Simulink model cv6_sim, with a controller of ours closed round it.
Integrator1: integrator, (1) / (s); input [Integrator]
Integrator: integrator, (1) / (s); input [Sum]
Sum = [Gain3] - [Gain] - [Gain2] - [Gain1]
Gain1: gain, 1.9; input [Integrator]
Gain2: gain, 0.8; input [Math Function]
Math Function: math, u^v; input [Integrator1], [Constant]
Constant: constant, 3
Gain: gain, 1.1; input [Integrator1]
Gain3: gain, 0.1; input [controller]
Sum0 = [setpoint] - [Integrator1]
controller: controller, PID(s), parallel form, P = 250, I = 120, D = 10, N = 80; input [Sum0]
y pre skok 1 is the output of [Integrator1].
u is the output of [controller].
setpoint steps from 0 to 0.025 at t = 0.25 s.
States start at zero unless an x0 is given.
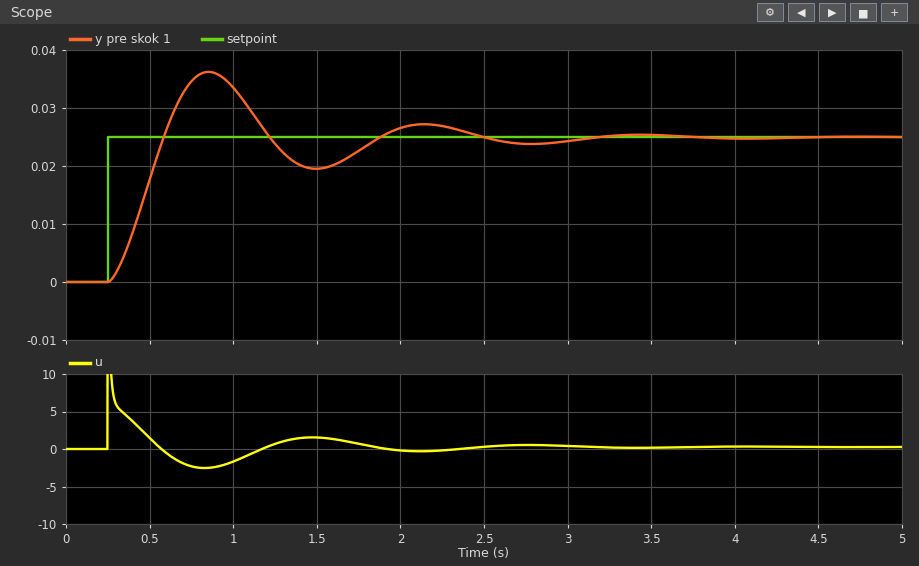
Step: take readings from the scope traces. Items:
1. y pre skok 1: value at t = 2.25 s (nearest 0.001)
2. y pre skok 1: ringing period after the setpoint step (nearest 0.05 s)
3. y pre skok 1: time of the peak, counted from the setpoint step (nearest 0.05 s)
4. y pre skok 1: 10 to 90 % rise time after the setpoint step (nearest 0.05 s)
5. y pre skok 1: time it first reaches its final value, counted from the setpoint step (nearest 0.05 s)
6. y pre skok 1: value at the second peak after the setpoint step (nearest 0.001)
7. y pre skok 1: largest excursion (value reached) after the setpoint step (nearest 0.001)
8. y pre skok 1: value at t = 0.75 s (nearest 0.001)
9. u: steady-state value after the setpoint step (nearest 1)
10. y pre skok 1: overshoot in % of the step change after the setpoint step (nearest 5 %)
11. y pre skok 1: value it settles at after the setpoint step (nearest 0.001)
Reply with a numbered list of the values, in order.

1. 0.027
2. 1.30 s
3. 0.60 s
4. 0.25 s
5. 0.35 s
6. 0.027
7. 0.036
8. 0.035
9. 0
10. 45 %
11. 0.025
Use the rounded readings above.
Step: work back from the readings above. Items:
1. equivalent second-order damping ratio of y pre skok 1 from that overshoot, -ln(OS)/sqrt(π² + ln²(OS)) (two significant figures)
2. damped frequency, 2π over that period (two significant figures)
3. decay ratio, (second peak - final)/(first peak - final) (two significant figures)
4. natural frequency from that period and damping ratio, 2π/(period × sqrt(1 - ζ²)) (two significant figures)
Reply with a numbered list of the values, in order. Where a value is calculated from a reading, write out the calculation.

1. ln(0.45) = -0.799; 0.799 / sqrt(9.870 + 0.638) = 0.25
2. 2π / 1.3 = 4.8 rad/s
3. (0.027 - 0.025) / (0.036 - 0.025) = 0.18
4. 2π / (1.3 × sqrt(1 - 0.25²)) = 5.0 rad/s
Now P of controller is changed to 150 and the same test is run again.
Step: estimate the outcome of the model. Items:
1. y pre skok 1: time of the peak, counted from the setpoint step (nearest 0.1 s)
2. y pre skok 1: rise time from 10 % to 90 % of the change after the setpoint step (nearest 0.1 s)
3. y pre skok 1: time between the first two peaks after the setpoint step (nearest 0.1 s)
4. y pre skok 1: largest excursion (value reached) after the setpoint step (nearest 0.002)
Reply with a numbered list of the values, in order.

1. 0.8 s
2. 0.3 s
3. 1.7 s
4. 0.036
